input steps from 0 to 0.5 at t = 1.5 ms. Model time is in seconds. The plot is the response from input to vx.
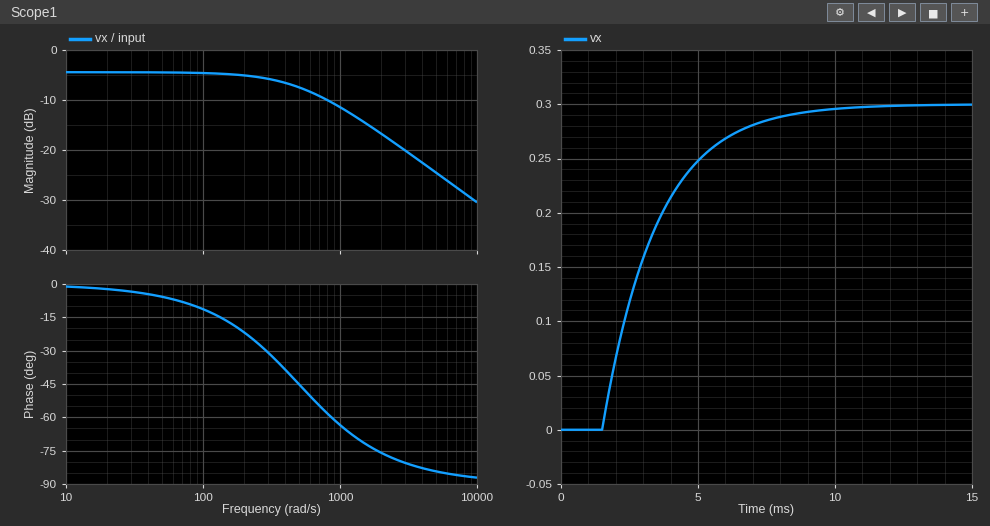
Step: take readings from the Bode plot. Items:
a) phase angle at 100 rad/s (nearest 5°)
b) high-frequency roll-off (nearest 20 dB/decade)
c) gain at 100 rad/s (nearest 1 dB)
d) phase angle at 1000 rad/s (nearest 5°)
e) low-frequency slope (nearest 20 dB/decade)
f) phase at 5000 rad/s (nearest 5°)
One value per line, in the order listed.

-10°
-20 dB/decade
-5 dB
-65°
0 dB/decade
-85°
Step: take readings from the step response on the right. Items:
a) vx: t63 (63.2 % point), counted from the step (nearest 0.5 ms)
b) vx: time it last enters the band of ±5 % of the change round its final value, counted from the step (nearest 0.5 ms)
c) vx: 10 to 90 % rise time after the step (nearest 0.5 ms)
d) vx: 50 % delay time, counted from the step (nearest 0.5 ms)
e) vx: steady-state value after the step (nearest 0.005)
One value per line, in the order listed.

2.0 ms
6.0 ms
4.5 ms
1.5 ms
0.300
